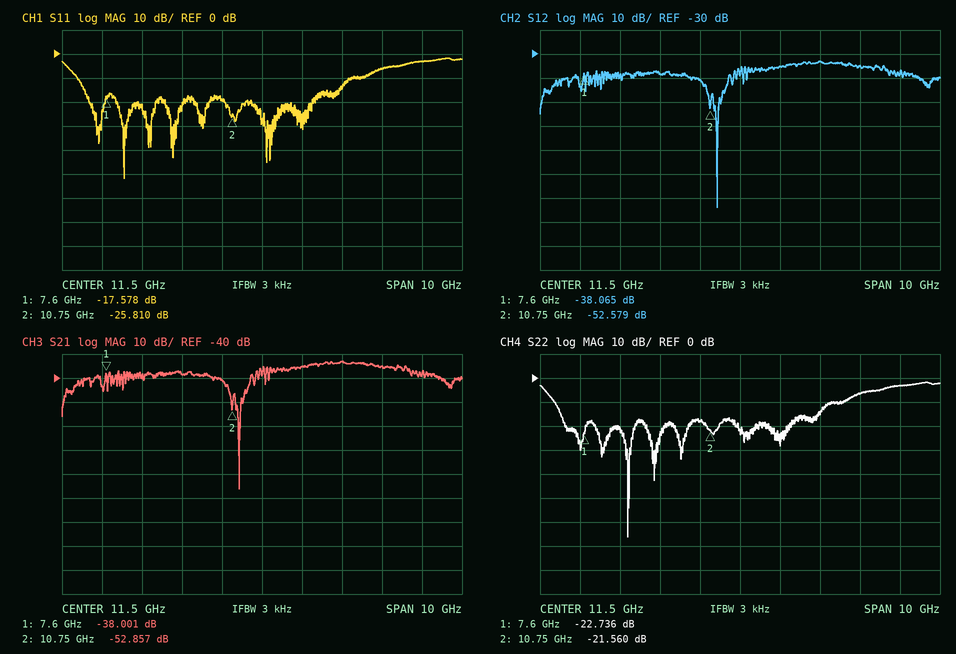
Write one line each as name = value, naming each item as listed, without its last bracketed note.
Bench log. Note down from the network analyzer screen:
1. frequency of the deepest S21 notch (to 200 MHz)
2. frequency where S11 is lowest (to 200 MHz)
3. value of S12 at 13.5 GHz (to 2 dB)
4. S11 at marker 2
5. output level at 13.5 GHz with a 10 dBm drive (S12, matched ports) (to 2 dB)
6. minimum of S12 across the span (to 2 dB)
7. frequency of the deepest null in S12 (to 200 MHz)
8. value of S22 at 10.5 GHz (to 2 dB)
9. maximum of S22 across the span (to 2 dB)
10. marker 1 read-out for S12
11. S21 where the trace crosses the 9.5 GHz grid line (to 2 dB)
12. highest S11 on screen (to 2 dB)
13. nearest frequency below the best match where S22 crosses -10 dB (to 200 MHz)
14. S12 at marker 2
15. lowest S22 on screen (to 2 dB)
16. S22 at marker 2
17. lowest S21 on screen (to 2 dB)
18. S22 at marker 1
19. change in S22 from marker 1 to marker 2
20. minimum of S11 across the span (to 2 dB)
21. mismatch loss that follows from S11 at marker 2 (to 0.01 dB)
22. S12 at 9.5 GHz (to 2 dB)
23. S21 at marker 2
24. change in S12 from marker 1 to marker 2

frequency of the deepest S21 notch = 11.0 GHz
frequency where S11 is lowest = 8.0 GHz
value of S12 at 13.5 GHz = -34 dB
S11 at marker 2 = -25.810 dB
output level at 13.5 GHz with a 10 dBm drive (S12, matched ports) = -24 dBm
minimum of S12 across the span = -94 dB
frequency of the deepest null in S12 = 11.0 GHz
value of S22 at 10.5 GHz = -18 dB
maximum of S22 across the span = -2 dB
marker 1 read-out for S12 = -38.065 dB
S21 where the trace crosses the 9.5 GHz grid line = -38 dB
highest S11 on screen = -2 dB
nearest frequency below the best match where S22 crosses -10 dB = 6.8 GHz
S12 at marker 2 = -52.579 dB
lowest S22 on screen = -66 dB
S22 at marker 2 = -21.560 dB
lowest S21 on screen = -86 dB
S22 at marker 1 = -22.736 dB
change in S22 from marker 1 to marker 2 = 1.176 dB
minimum of S11 across the span = -52 dB
mismatch loss that follows from S11 at marker 2 = 0.01 dB
S12 at 9.5 GHz = -38 dB
S21 at marker 2 = -52.857 dB
change in S12 from marker 1 to marker 2 = -14.514 dB
